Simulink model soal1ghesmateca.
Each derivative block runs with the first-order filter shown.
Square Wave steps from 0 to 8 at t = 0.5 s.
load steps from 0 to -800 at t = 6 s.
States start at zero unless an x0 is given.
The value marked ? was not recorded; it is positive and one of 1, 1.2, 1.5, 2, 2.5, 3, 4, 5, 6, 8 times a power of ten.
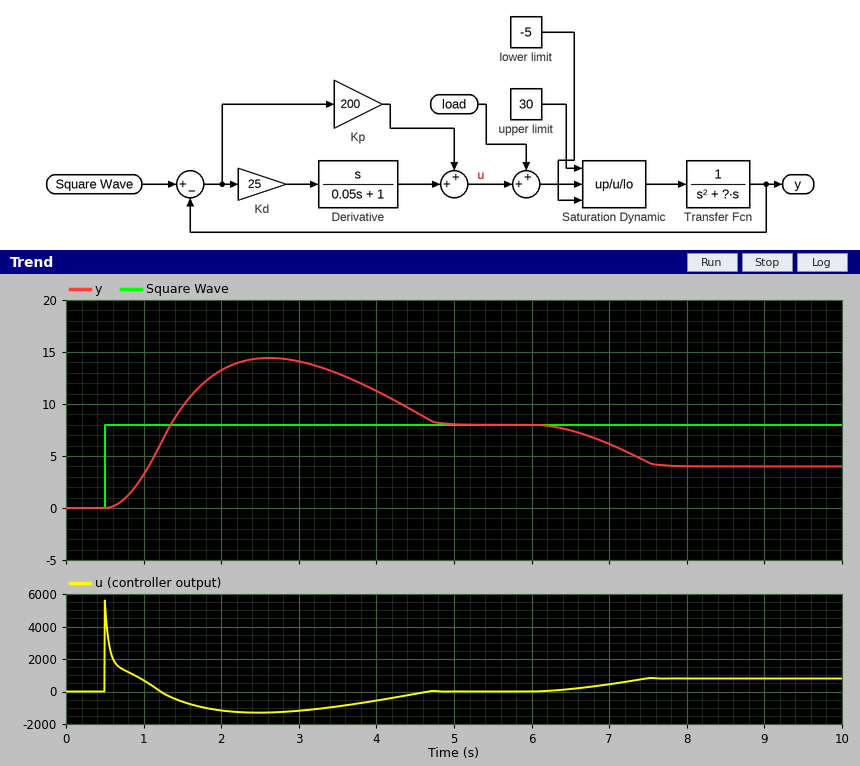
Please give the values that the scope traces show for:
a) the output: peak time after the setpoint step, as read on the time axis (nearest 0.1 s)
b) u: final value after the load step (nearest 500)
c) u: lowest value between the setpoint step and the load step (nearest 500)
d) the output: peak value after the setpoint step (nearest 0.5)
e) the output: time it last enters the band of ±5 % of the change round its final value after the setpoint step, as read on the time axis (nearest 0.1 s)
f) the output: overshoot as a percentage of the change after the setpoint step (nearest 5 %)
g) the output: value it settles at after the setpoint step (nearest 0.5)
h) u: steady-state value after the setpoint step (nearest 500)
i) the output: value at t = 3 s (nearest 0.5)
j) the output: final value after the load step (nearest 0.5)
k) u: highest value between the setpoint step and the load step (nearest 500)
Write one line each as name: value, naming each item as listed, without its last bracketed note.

the output: peak time after the setpoint step, as read on the time axis: 2.6 s
u: final value after the load step: 1000
u: lowest value between the setpoint step and the load step: -1500
the output: peak value after the setpoint step: 14.5
the output: time it last enters the band of ±5 % of the change round its final value after the setpoint step, as read on the time axis: 4.7 s
the output: overshoot as a percentage of the change after the setpoint step: 80 %
the output: value it settles at after the setpoint step: 8.0
u: steady-state value after the setpoint step: 0
the output: value at t = 3 s: 14.0
the output: final value after the load step: 4.0
u: highest value between the setpoint step and the load step: 5500
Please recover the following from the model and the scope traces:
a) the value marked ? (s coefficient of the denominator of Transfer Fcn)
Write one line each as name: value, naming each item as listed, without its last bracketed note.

the value marked ?: 1
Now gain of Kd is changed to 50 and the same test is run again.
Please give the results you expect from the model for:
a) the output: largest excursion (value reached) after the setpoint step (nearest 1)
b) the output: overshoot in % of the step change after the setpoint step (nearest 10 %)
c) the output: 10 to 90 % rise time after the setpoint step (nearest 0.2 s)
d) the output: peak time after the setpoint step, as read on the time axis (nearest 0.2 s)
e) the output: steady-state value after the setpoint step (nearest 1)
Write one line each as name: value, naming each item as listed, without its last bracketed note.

the output: largest excursion (value reached) after the setpoint step: 12
the output: overshoot in % of the step change after the setpoint step: 50 %
the output: 10 to 90 % rise time after the setpoint step: 0.6 s
the output: peak time after the setpoint step, as read on the time axis: 2.4 s
the output: steady-state value after the setpoint step: 8
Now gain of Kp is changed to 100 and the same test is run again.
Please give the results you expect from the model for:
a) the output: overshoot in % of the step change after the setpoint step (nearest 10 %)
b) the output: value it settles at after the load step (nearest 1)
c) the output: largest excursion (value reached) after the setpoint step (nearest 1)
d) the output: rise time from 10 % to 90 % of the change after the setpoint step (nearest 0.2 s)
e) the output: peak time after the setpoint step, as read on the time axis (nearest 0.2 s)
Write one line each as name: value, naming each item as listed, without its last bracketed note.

the output: overshoot in % of the step change after the setpoint step: 50 %
the output: value it settles at after the load step: 0
the output: largest excursion (value reached) after the setpoint step: 12
the output: rise time from 10 % to 90 % of the change after the setpoint step: 0.6 s
the output: peak time after the setpoint step, as read on the time axis: 2.4 s
